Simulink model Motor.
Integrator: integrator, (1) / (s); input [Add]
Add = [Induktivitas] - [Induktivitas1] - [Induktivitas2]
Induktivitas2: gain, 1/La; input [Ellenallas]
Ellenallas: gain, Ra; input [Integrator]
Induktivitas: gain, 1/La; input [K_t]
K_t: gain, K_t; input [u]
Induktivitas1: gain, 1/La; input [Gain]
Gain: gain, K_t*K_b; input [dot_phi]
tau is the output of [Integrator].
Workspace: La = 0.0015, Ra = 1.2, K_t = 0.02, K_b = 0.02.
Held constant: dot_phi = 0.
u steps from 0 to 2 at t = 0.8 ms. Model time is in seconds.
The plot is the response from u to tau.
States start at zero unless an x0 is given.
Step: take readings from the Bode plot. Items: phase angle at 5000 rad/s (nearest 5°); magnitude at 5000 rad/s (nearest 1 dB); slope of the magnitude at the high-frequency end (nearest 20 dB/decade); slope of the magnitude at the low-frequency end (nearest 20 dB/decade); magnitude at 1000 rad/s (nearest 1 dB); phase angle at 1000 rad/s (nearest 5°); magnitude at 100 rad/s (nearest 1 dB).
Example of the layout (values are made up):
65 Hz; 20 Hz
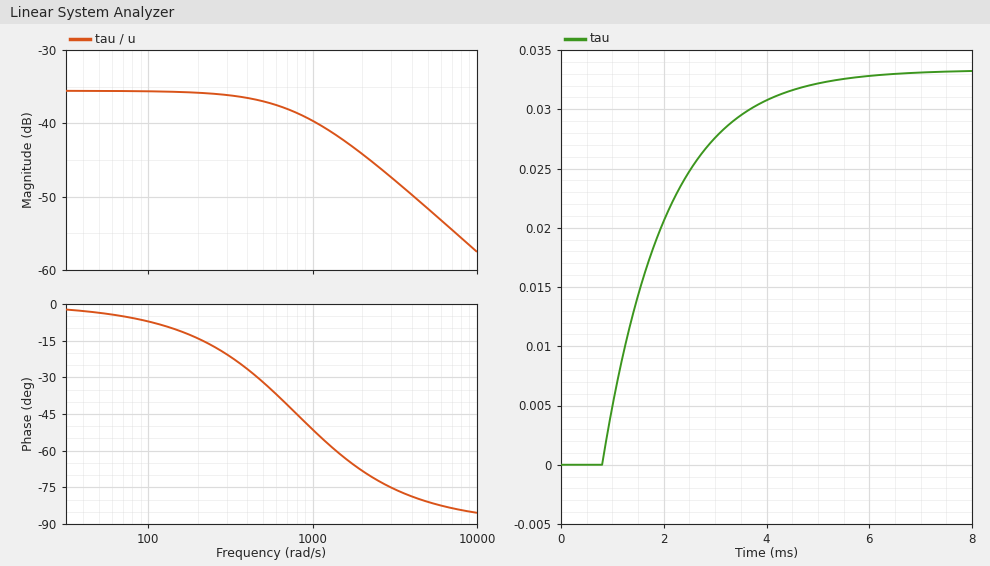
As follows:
-80°; -52 dB; -20 dB/decade; 0 dB/decade; -40 dB; -50°; -36 dB
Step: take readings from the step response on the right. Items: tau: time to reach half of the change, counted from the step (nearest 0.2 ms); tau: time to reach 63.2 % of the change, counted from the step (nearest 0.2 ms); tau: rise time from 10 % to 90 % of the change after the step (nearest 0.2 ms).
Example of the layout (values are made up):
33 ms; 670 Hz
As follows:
0.8 ms; 1.2 ms; 2.8 ms
